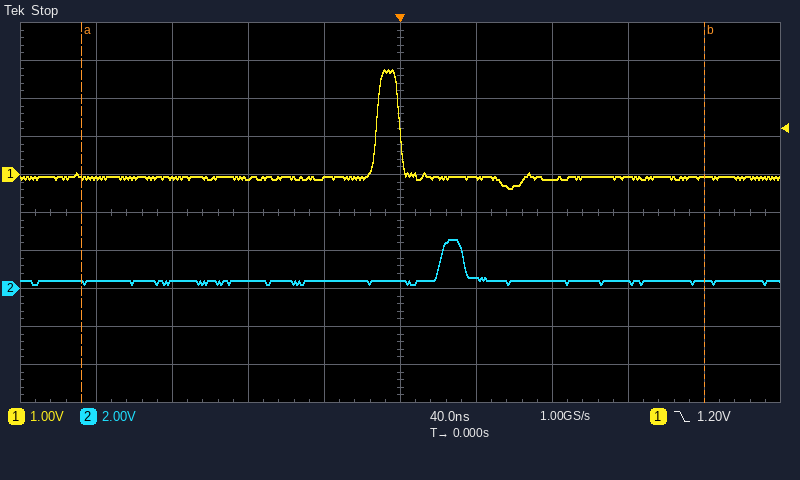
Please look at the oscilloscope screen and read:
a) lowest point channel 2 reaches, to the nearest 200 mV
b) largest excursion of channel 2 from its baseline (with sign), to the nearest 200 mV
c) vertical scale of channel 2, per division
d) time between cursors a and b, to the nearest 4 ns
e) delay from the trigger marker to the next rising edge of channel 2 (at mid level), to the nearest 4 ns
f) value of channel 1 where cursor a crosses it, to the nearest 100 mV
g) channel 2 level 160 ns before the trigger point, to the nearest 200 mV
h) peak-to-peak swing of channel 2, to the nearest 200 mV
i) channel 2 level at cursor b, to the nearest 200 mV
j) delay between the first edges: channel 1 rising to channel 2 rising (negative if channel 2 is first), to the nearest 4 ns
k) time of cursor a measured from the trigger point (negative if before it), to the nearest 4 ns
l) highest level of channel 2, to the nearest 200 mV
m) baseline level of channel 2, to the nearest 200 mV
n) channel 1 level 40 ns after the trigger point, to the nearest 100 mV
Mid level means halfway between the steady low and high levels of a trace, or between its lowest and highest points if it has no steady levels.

200 mV
+2.2 V
2 V
328 ns
20 ns
-100 mV
400 mV
2.4 V
400 mV
+32 ns
-168 ns
2.6 V
400 mV
-100 mV
